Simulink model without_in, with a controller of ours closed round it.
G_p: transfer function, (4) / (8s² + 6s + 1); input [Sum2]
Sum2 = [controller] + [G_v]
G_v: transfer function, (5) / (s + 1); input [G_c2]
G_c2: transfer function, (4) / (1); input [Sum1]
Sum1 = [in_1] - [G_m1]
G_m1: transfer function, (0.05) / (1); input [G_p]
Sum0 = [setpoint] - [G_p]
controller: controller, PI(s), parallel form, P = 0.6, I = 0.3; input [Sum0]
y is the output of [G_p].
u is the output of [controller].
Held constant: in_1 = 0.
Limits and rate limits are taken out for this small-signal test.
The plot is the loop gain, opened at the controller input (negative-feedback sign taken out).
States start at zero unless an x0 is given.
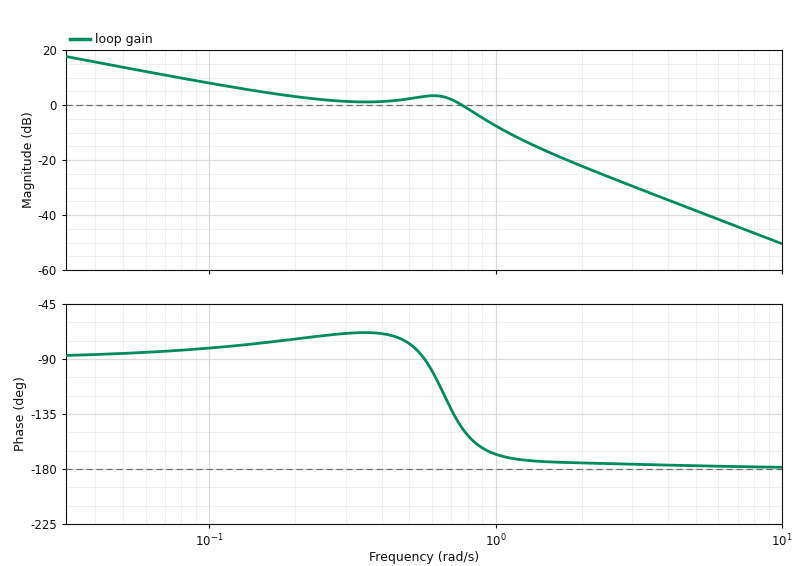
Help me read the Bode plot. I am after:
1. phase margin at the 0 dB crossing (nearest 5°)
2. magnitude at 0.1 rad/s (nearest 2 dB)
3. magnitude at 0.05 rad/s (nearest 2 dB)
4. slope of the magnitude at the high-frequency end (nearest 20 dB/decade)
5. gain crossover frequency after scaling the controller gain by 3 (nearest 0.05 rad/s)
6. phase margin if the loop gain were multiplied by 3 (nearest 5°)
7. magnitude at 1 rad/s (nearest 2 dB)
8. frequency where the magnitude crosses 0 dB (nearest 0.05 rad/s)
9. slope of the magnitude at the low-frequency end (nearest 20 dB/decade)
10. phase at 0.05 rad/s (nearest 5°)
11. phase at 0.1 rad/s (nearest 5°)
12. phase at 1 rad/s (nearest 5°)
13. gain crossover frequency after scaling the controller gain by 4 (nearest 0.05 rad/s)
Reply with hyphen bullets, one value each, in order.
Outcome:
- 35°
- 8 dB
- 14 dB
- -40 dB/decade
- 1.10 rad/s
- 10°
- -8 dB
- 0.75 rad/s
- -20 dB/decade
- -85°
- -80°
- -170°
- 1.20 rad/s
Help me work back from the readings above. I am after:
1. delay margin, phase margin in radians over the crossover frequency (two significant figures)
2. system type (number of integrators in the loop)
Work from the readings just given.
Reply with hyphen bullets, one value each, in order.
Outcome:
- 0.81 s
- 1
